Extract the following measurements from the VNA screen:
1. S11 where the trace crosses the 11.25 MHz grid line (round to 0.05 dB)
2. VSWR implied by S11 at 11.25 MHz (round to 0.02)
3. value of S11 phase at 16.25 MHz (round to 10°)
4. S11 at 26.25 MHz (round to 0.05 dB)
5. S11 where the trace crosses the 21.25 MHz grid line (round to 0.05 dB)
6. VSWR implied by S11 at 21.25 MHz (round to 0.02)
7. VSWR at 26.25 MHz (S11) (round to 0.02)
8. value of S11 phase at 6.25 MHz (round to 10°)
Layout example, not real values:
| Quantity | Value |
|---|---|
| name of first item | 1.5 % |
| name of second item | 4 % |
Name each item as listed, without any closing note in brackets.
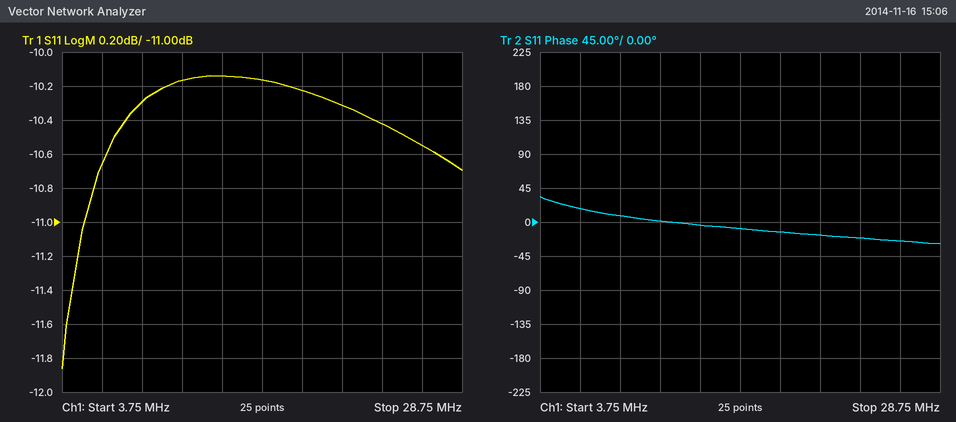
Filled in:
| Quantity | Value |
|---|---|
| S11 where the trace crosses the 11.25 MHz grid line | -10.15 dB |
| VSWR implied by S11 at 11.25 MHz | 1.90 |
| value of S11 phase at 16.25 MHz | -10° |
| S11 at 26.25 MHz | -10.55 dB |
| S11 where the trace crosses the 21.25 MHz grid line | -10.30 dB |
| VSWR implied by S11 at 21.25 MHz | 1.88 |
| VSWR at 26.25 MHz (S11) | 1.84 |
| value of S11 phase at 6.25 MHz | 20° |
